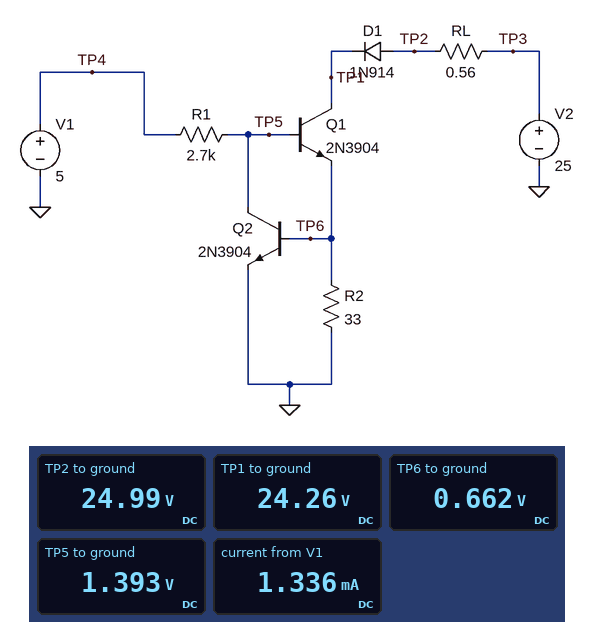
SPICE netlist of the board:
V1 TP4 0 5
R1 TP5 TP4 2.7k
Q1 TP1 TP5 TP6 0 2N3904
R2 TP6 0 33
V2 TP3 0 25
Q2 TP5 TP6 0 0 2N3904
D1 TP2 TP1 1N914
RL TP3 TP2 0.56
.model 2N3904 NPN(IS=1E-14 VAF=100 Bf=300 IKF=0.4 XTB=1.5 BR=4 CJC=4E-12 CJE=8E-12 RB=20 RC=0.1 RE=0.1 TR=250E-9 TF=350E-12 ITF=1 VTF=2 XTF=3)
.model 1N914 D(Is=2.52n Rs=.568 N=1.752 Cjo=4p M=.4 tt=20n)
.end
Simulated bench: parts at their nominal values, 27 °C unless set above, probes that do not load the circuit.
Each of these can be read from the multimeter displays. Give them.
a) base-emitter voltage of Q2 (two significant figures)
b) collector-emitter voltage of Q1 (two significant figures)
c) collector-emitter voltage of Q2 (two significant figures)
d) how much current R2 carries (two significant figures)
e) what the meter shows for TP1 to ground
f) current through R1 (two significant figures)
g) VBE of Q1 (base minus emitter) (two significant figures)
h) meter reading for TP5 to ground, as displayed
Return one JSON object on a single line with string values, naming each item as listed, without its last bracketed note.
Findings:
{"base-emitter voltage of Q2": "660 mV", "collector-emitter voltage of Q1": "24 V", "collector-emitter voltage of Q2": "1.4 V", "how much current R2 carries": "20 mA", "what the meter shows for TP1 to ground": "24.26 V", "current through R1": "1.3 mA", "VBE of Q1 (base minus emitter)": "730 mV", "meter reading for TP5 to ground, as displayed": "1.393 V"}
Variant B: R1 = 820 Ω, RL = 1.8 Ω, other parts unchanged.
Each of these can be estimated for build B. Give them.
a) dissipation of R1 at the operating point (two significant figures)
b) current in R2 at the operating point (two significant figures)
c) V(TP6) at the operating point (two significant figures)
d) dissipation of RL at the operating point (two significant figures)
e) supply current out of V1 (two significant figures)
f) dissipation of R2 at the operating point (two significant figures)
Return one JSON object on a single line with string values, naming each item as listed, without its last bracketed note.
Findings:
{"dissipation of R1 at the operating point": "16 mW", "current in R2 at the operating point": "21 mA", "V(TP6) at the operating point": "690 mV", "dissipation of RL at the operating point": "790 µW", "supply current out of V1": "4.4 mA", "dissipation of R2 at the operating point": "15 mW"}
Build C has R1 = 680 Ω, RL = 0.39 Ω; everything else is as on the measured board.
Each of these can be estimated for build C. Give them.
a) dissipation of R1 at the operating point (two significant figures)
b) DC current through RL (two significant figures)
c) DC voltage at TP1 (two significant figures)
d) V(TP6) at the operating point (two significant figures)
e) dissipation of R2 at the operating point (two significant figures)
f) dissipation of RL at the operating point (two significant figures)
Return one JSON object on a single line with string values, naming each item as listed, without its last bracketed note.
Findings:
{"dissipation of R1 at the operating point": "19 mW", "DC current through RL": "21 mA", "DC voltage at TP1": "24 V", "V(TP6) at the operating point": "700 mV", "dissipation of R2 at the operating point": "15 mW", "dissipation of RL at the operating point": "170 µW"}
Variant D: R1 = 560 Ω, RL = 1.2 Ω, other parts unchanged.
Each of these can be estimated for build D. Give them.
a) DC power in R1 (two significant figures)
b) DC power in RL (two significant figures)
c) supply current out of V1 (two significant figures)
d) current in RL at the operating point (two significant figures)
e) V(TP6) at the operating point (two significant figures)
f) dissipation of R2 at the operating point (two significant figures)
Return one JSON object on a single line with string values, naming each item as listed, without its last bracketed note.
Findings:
{"DC power in R1": "23 mW", "DC power in RL": "540 µW", "supply current out of V1": "6.4 mA", "current in RL at the operating point": "21 mA", "V(TP6) at the operating point": "700 mV", "dissipation of R2 at the operating point": "15 mW"}
